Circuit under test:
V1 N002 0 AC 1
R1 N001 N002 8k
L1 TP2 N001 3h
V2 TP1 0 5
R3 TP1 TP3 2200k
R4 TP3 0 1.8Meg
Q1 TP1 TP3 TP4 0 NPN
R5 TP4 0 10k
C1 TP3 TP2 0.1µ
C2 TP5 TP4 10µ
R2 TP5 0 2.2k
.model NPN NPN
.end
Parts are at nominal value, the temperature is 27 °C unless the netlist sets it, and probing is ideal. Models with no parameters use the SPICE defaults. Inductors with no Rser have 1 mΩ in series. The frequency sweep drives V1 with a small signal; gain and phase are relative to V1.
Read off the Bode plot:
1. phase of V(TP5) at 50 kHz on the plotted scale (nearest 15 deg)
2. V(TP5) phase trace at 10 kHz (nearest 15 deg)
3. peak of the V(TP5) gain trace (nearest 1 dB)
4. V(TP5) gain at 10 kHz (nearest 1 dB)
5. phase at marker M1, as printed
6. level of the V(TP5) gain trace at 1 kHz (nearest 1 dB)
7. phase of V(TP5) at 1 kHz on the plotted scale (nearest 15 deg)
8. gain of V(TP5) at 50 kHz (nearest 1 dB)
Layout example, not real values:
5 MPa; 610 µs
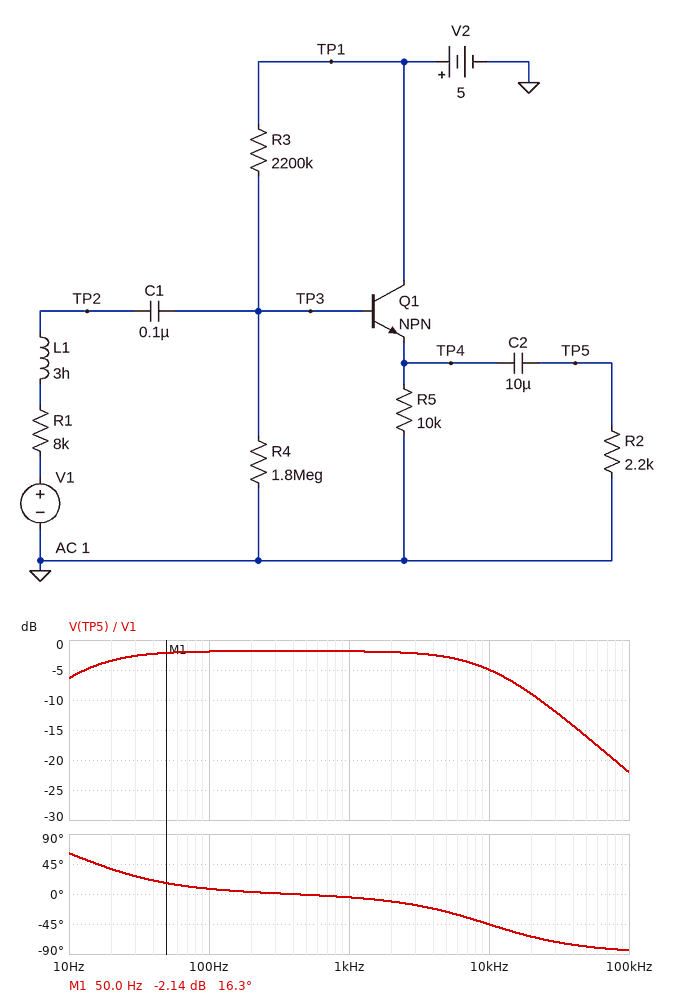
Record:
-75 deg; -45 deg; -2 dB; -5 dB; 16.3 deg; -2 dB; 0 deg; -16 dB
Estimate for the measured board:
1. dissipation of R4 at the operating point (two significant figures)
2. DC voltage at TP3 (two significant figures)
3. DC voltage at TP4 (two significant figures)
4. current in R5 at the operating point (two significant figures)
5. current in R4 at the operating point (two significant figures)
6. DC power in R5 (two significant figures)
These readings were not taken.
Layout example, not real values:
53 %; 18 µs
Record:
1.2 µW; 1.5 V; 780 mV; 78 µA; 830 nA; 61 µW
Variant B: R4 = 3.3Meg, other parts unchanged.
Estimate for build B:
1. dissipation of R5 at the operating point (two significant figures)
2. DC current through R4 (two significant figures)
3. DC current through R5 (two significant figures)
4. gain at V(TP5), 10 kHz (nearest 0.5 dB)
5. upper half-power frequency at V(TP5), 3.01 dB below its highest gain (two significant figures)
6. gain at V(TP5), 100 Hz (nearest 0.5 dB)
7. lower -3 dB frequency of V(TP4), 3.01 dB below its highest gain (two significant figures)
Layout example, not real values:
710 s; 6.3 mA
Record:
98 µW; 520 nA; 99 µA; -4.5 dB; 10 kHz; -1.5 dB; 9.1 Hz
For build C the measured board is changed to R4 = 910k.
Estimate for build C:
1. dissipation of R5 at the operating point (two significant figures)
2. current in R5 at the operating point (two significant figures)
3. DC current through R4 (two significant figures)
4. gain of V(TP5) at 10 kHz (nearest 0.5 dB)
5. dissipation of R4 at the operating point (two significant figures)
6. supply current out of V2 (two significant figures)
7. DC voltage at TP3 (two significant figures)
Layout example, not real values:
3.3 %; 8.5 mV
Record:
22 µW; 47 µA; 1.3 µA; -6.0 dB; 1.5 µW; 48 µA; 1.2 V
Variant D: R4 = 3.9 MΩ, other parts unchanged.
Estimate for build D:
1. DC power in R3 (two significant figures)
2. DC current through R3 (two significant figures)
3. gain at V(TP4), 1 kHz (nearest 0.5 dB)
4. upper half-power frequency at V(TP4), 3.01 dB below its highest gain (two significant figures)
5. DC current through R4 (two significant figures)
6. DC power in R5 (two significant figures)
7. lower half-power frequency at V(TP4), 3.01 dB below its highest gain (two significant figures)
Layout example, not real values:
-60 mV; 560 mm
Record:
4.8 µW; 1.5 µA; -1.5 dB; 10 kHz; 450 nA; 110 µW; 9.1 Hz
